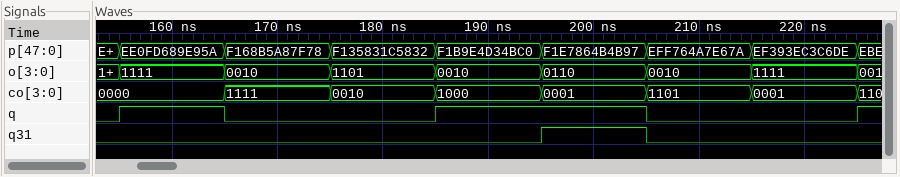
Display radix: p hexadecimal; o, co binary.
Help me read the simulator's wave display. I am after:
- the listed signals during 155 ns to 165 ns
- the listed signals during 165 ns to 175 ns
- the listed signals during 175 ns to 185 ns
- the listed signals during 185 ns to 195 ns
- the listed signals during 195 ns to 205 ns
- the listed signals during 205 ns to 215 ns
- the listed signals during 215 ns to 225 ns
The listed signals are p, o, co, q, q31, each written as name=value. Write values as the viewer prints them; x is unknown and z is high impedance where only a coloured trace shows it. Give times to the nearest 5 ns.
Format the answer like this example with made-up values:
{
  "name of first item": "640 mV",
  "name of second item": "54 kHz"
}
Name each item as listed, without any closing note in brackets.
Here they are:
{
  "the listed signals during 155 ns to 165 ns": "p=EE0FD689E95A, o=1111, co=0000, q=1, q31=0",
  "the listed signals during 165 ns to 175 ns": "p=F168B5A87F78, o=0010, co=1111, q=0, q31=0",
  "the listed signals during 175 ns to 185 ns": "p=F135831C5832, o=1101, co=0010, q=0, q31=0",
  "the listed signals during 185 ns to 195 ns": "p=F1B9E4D34BC0, o=0010, co=1000, q=1, q31=0",
  "the listed signals during 195 ns to 205 ns": "p=F1E7864B4B97, o=0110, co=0001, q=1, q31=1",
  "the listed signals during 205 ns to 215 ns": "p=EFF764A7E67A, o=0010, co=1101, q=0, q31=0",
  "the listed signals during 215 ns to 225 ns": "p=EF393EC3C6DE, o=1111, co=0001, q=0, q31=0"
}
